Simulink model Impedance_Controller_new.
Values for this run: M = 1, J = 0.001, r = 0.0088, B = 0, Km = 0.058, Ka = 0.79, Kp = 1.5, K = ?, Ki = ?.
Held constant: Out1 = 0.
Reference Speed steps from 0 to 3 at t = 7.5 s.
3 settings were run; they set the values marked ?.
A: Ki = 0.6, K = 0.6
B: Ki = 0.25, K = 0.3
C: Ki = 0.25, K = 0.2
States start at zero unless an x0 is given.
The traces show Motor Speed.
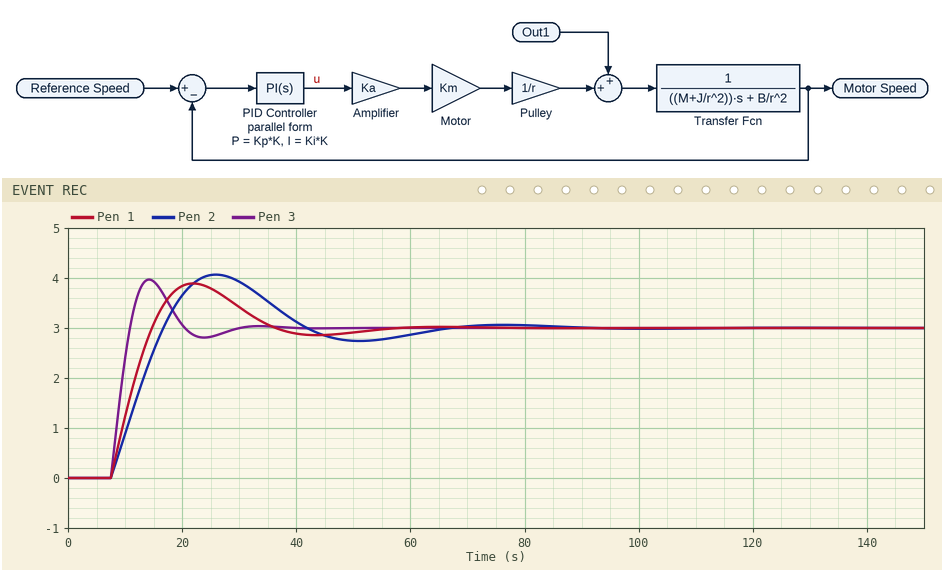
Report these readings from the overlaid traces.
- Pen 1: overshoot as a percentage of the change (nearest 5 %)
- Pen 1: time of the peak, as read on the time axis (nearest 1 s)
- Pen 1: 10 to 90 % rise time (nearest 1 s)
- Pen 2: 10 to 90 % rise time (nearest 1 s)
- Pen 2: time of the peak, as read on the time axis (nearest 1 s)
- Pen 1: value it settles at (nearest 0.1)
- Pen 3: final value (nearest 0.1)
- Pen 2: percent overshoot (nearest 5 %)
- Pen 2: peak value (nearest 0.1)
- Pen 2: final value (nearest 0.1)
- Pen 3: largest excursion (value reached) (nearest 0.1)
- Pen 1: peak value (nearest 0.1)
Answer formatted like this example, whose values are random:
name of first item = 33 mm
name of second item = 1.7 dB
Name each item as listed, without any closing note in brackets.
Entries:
Pen 1: overshoot as a percentage of the change = 30 %
Pen 1: time of the peak, as read on the time axis = 22 s
Pen 1: 10 to 90 % rise time = 6 s
Pen 2: 10 to 90 % rise time = 7 s
Pen 2: time of the peak, as read on the time axis = 26 s
Pen 1: value it settles at = 3.0
Pen 3: final value = 3.0
Pen 2: percent overshoot = 35 %
Pen 2: peak value = 4.1
Pen 2: final value = 3.0
Pen 3: largest excursion (value reached) = 4.0
Pen 1: peak value = 3.9
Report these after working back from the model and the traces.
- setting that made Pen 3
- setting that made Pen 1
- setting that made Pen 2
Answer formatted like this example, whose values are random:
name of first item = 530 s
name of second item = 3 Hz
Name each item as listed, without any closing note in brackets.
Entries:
setting that made Pen 3 = A
setting that made Pen 1 = B
setting that made Pen 2 = C
